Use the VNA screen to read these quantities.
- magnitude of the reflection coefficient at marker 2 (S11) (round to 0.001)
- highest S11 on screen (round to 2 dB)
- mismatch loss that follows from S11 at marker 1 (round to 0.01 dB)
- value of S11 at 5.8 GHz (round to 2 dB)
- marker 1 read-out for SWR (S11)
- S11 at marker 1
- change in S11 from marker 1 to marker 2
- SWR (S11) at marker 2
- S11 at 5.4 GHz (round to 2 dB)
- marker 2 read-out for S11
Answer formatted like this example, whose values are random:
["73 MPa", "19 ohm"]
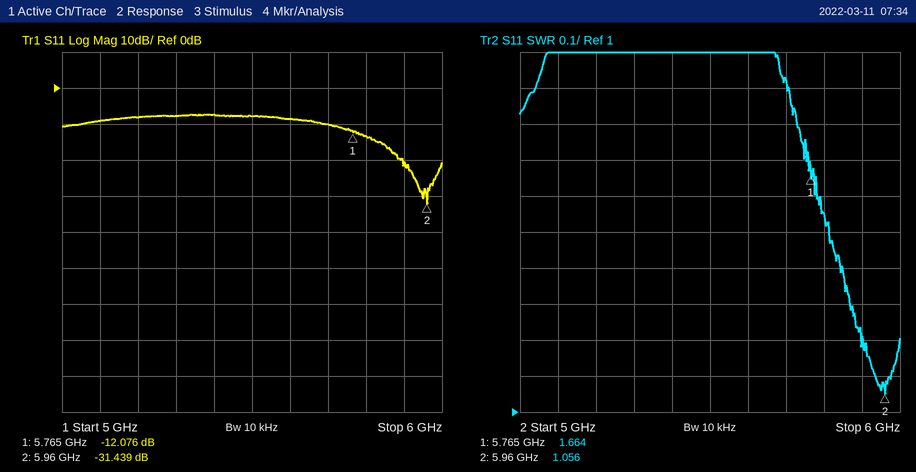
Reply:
["0.027", "-8 dB", "0.28 dB", "-14 dB", "1.664", "-12.076 dB", "-19.363 dB", "1.056", "-8 dB", "-31.439 dB"]
